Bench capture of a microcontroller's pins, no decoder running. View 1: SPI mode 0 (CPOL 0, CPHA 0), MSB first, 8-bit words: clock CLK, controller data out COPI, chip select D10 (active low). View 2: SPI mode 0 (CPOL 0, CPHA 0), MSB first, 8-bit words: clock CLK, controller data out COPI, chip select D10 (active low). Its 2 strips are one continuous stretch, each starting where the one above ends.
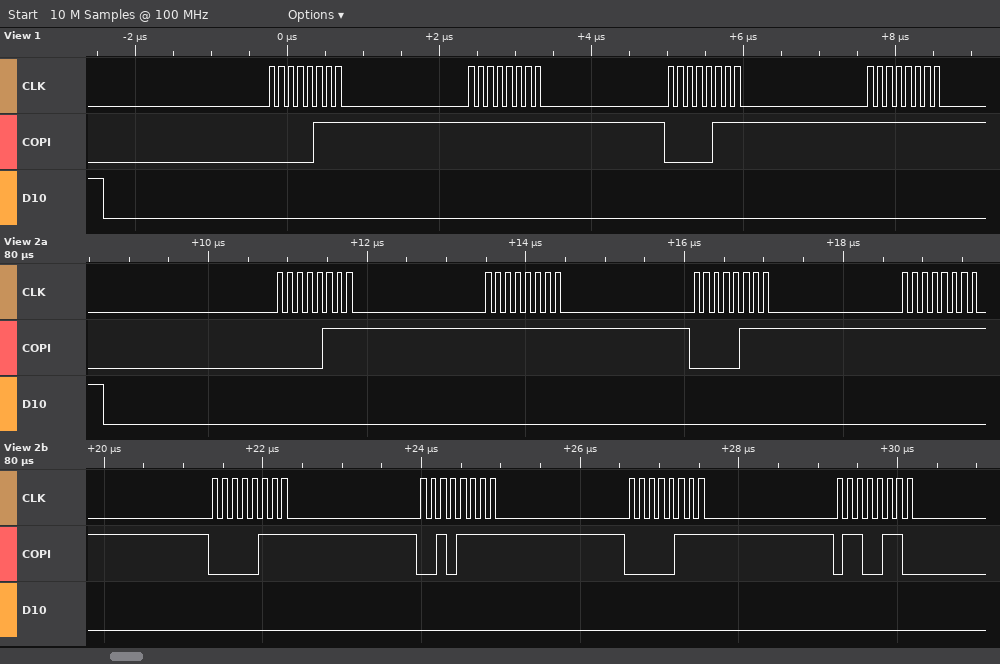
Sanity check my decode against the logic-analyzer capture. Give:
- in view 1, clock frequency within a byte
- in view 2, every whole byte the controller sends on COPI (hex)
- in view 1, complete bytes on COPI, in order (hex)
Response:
8 MHz
0x07 0xFF 0x07 0xFF 0x07 0x2F 0x07 0x66
0x07 0xFF 0x07 0xFF
